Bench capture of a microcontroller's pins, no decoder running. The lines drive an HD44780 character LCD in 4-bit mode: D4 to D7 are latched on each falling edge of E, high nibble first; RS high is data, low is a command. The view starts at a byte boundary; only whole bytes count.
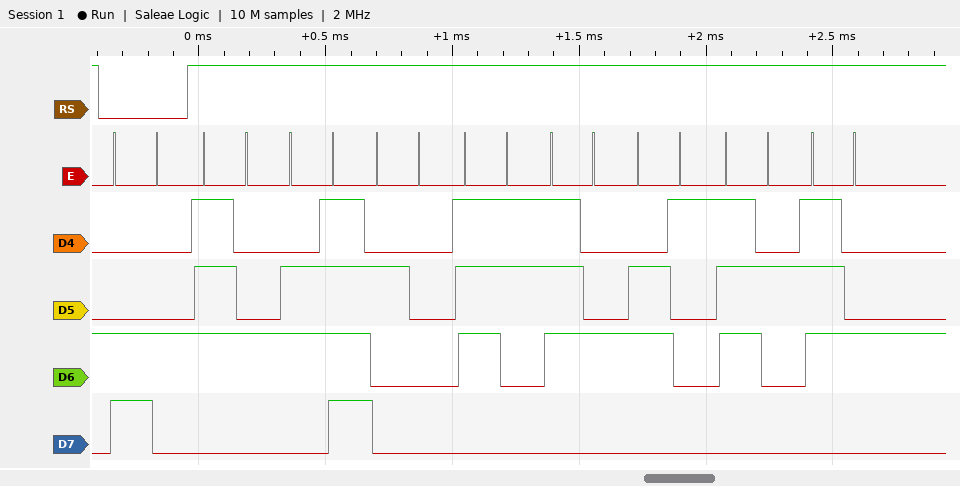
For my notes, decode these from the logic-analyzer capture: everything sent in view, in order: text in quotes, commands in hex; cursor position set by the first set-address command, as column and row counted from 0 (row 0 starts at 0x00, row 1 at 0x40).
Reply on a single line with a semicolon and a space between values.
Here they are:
0xC4 "to start"; column 4, row 1
